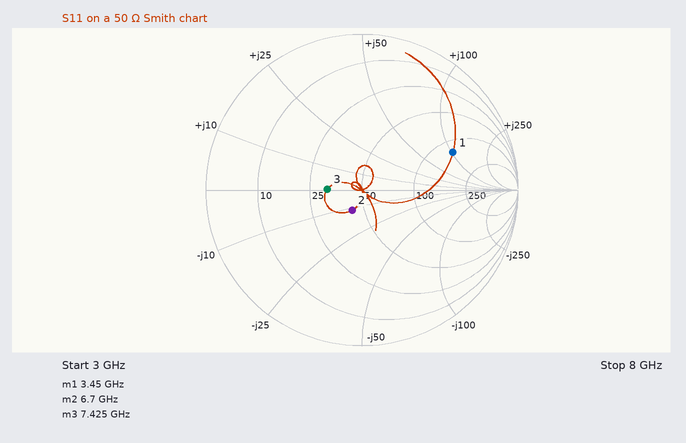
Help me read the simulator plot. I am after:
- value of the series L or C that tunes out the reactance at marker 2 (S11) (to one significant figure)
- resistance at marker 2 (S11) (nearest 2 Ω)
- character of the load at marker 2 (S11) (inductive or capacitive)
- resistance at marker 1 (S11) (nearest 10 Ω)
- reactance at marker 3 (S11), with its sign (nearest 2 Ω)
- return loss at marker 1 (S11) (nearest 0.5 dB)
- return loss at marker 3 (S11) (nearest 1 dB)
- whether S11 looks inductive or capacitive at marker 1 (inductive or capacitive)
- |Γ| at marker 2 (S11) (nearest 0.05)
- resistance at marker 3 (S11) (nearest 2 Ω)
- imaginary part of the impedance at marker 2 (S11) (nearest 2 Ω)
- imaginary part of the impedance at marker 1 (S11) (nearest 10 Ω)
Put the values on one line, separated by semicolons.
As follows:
300 pH; 42 Ω; capacitive; 130 Ω; 0 Ω; 4.0 dB; 13 dB; inductive; 0.15; 32 Ω; -12 Ω; +100 Ω
